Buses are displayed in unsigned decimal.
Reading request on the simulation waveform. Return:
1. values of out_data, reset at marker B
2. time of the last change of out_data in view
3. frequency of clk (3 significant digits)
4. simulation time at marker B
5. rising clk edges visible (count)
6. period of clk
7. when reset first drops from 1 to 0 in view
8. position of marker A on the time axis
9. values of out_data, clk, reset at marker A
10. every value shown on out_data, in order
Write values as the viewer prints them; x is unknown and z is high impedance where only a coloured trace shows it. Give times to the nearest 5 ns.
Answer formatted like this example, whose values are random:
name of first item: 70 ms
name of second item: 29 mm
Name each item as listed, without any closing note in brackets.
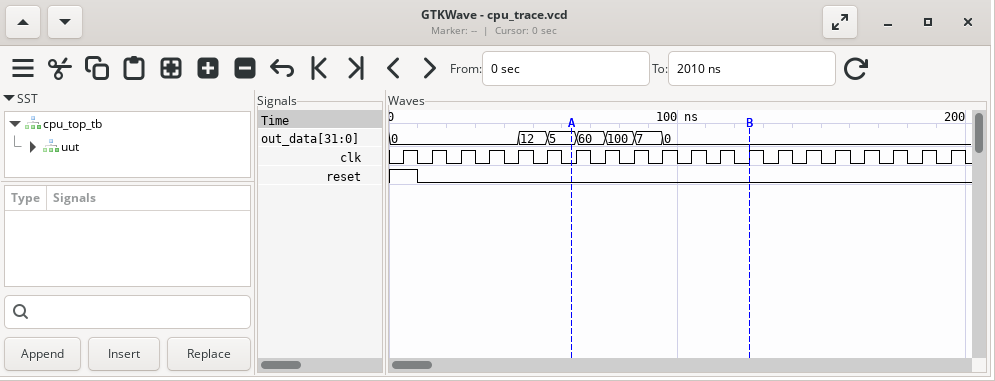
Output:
values of out_data, reset at marker B: out_data=0, reset=0
time of the last change of out_data in view: 95 ns
frequency of clk: 100 MHz
simulation time at marker B: 125 ns
rising clk edges visible: 20
period of clk: 10 ns
when reset first drops from 1 to 0 in view: 10 ns
position of marker A on the time axis: 65 ns
values of out_data, clk, reset at marker A: out_data=5, clk=0, reset=0
every value shown on out_data, in order: 0, 12, 5, 60, 100, 7, 0
